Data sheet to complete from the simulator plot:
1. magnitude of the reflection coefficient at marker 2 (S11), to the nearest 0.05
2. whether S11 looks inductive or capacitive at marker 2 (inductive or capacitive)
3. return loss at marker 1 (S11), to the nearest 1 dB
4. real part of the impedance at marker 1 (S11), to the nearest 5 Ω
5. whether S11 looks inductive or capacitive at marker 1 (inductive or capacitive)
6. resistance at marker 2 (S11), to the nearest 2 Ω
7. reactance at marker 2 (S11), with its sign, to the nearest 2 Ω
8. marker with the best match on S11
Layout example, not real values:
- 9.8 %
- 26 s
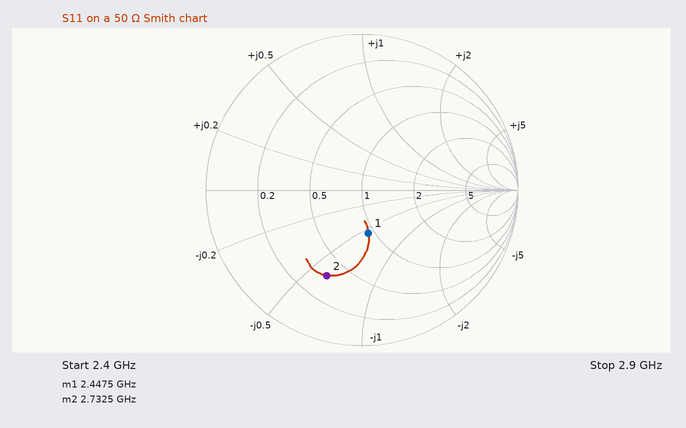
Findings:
- 0.60
- capacitive
- 11 dB
- 45 Ω
- capacitive
- 18 Ω
- -30 Ω
- marker 1
